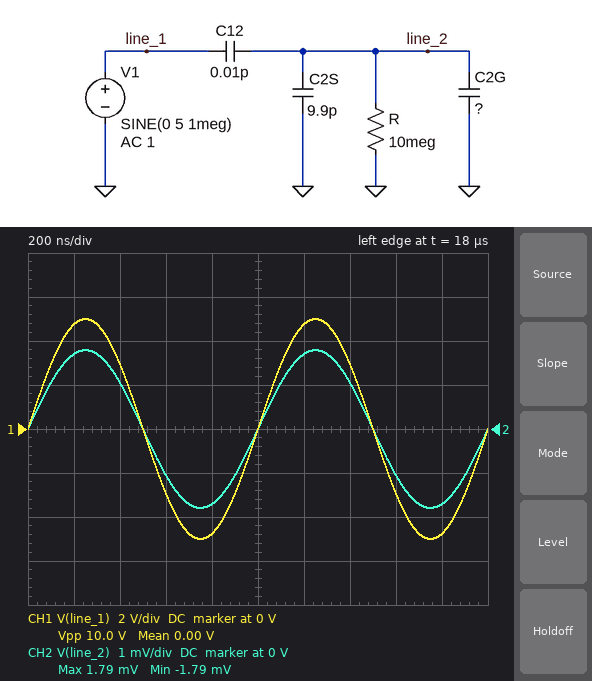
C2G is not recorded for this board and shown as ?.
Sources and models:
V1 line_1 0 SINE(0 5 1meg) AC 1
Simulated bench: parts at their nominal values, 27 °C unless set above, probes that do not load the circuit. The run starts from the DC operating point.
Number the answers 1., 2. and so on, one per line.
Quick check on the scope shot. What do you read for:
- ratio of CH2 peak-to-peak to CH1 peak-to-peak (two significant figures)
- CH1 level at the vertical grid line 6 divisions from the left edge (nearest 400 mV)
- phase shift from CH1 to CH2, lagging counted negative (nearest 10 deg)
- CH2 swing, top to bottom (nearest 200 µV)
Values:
1. 0.00036
2. 4.8 V
3. 0 deg
4. 3.6 mV
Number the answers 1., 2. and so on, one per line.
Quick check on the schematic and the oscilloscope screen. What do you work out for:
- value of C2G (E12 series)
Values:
1. 18 pF
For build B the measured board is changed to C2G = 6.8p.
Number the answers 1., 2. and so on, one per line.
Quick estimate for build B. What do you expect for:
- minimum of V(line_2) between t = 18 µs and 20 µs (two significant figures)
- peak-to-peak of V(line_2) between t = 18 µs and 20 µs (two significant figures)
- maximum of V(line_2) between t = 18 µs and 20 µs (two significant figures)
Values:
1. -3.0 mV
2. 6.0 mV
3. 3.0 mV
